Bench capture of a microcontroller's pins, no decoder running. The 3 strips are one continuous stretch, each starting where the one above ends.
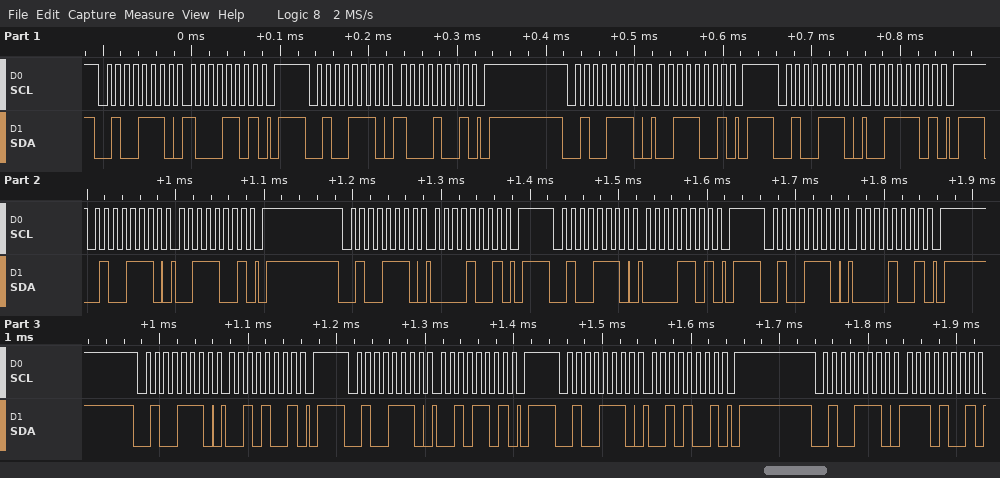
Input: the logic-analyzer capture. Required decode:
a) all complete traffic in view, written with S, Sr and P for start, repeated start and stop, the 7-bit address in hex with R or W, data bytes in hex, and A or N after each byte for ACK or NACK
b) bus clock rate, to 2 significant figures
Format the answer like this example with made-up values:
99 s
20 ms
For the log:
S 27W A 8D A P S 27W A 89 A P S 27W A 39 A P S 27W A 3D A P S 27W A 39 A P S 27W A 09 A P S 27W A 0D A P S 27W A 09 A P S 27W A 29 A P S 27W A 2D A P S 27W A 29 A P S 27W A E9 A
100 kHz
